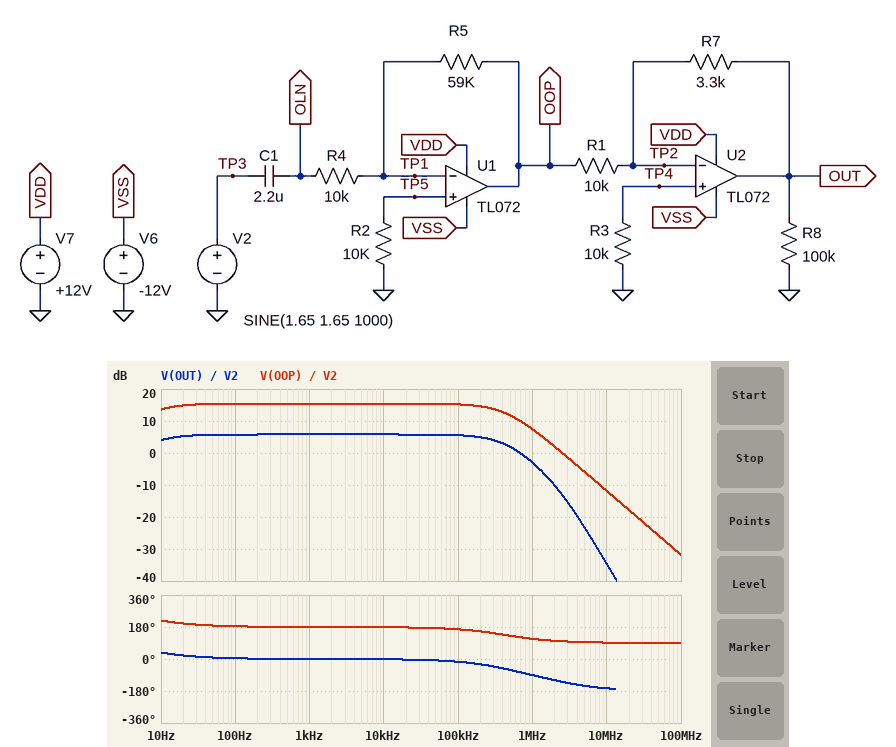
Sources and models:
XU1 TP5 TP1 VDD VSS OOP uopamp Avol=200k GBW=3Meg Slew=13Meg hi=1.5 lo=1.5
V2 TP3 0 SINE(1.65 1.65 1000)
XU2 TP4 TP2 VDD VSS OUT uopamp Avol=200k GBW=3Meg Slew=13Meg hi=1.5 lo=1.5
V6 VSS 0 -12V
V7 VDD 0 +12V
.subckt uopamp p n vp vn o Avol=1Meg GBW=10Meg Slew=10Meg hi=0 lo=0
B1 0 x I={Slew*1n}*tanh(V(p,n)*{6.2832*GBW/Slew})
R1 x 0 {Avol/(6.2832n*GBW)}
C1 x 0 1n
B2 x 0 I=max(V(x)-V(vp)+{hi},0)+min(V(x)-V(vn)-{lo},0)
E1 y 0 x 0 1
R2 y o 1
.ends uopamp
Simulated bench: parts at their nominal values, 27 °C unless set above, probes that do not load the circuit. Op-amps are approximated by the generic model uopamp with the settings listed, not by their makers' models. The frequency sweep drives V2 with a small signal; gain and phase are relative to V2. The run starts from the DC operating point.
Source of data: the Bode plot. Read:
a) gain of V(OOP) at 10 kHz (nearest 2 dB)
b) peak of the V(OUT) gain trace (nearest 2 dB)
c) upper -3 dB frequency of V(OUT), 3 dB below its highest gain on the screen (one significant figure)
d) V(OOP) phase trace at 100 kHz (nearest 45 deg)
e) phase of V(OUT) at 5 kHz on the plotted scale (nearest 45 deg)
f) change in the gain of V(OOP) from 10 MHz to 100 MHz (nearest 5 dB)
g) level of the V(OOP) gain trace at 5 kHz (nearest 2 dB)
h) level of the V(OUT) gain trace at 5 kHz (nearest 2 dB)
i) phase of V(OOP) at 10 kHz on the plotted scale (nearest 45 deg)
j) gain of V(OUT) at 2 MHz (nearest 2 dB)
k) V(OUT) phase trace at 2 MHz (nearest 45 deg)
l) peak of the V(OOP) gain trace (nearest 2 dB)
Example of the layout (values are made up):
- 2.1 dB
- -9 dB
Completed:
- 16 dB
- 6 dB
- 400 kHz
- 180 deg
- 0 deg
- -20 dB
- 16 dB
- 6 dB
- 180 deg
- -10 dB
- -135 deg
- 16 dB
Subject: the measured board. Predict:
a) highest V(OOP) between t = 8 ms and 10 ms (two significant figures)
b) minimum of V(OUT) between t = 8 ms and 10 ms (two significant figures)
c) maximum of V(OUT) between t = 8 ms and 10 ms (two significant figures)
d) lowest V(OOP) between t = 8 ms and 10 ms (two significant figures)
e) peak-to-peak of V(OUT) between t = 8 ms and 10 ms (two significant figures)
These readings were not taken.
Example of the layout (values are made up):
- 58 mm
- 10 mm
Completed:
- 9.8 V
- -3.2 V
- 3.2 V
- -9.7 V
- 6.4 V
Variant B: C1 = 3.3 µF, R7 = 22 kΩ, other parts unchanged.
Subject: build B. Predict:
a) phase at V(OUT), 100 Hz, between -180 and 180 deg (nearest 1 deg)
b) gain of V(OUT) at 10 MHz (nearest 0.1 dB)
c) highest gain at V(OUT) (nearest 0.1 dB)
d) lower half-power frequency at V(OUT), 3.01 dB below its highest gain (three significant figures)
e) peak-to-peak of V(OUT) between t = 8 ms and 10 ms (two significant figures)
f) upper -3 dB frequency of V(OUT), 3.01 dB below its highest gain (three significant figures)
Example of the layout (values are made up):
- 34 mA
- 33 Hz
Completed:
- 3 deg
- -25.6 dB
- 22.3 dB
- 4.82 Hz
- 21 V
- 371 kHz
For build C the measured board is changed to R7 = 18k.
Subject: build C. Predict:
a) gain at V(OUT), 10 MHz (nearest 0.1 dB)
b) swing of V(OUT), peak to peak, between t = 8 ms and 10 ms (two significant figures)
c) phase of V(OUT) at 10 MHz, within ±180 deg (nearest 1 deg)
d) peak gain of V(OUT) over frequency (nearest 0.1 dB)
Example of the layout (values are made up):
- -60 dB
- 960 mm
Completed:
- -26.2 dB
- 21 V
- -171 deg
- 20.5 dB
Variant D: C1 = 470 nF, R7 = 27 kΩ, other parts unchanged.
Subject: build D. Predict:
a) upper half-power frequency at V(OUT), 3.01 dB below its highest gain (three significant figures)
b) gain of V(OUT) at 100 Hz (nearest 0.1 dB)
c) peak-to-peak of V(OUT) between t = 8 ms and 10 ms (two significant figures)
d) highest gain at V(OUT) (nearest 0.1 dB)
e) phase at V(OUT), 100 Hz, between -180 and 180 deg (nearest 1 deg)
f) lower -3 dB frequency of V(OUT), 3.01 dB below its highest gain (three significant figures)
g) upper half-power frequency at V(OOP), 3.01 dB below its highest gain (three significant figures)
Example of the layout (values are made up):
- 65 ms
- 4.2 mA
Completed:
- 357 kHz
- 23.6 dB
- 21 V
- 24.0 dB
- 19 deg
- 33.9 Hz
- 435 kHz
